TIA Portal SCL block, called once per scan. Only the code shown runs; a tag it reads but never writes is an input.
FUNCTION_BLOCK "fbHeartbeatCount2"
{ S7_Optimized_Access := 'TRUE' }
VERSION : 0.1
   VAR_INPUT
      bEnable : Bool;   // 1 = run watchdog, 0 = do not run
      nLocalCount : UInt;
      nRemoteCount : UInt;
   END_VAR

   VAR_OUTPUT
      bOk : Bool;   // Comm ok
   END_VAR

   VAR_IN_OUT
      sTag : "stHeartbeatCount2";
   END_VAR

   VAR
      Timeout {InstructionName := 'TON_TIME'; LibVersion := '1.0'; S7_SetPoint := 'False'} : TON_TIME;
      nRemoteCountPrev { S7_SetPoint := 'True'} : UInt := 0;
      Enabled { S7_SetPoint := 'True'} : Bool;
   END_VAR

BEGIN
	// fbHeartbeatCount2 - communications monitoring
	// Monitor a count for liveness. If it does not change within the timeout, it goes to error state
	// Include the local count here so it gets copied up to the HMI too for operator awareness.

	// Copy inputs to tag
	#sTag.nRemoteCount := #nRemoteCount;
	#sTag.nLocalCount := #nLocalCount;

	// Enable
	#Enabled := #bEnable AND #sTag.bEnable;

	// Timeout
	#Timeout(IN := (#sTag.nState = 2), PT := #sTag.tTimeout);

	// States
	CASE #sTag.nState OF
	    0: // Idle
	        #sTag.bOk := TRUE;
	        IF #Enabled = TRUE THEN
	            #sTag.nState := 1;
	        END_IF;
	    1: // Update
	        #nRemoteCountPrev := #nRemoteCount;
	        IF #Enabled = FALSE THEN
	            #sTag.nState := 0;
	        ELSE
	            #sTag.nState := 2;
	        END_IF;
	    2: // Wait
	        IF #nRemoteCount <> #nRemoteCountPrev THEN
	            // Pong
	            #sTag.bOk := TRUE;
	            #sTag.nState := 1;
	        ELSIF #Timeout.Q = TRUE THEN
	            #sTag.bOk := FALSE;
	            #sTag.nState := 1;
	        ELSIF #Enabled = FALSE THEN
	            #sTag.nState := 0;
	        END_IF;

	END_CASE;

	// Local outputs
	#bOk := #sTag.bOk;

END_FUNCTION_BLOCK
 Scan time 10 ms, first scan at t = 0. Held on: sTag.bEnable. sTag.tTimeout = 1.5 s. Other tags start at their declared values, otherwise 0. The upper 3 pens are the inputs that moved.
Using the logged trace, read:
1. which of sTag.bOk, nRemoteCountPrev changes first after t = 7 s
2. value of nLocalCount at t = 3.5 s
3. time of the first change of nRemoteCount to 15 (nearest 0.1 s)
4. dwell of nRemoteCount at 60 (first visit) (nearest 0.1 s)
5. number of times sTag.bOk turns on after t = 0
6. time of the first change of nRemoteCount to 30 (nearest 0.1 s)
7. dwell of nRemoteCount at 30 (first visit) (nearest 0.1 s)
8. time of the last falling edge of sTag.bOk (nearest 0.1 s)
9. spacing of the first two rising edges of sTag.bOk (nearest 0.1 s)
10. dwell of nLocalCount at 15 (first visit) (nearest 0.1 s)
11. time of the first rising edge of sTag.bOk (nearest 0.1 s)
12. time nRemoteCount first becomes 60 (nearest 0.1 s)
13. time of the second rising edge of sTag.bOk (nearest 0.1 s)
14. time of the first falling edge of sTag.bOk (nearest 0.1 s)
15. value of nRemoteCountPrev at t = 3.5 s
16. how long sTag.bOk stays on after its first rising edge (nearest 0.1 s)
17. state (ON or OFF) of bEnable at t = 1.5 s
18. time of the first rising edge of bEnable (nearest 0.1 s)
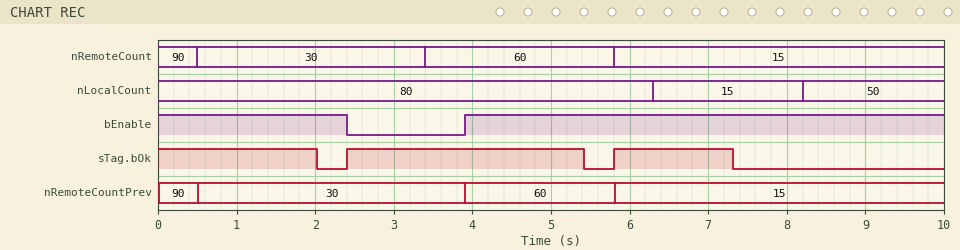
sTag.bOk
80
5.8 s
2.4 s
2
0.5 s
2.9 s
7.3 s
3.4 s
1.9 s
2.4 s
3.4 s
5.8 s
2.0 s
30
3.0 s
ON
3.9 s
